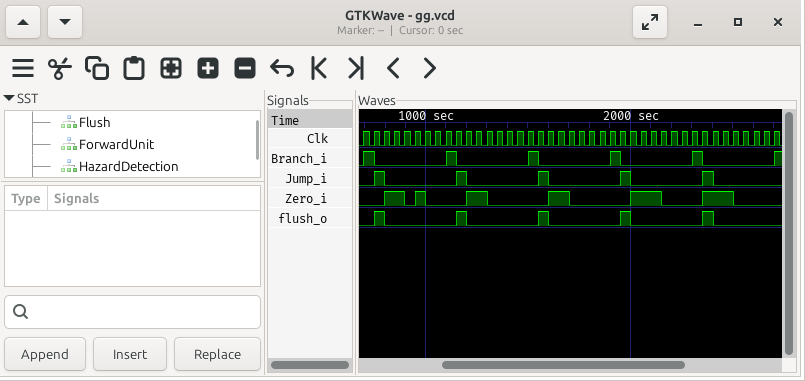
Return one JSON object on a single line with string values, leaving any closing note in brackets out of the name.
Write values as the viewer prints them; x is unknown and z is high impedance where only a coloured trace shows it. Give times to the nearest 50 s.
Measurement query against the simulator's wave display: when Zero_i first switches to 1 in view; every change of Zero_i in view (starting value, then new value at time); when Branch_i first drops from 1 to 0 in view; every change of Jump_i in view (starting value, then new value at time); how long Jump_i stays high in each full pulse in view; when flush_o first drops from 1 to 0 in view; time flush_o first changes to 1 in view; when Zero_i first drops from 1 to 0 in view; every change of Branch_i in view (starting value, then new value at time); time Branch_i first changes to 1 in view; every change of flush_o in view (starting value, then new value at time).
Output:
{"when Zero_i first switches to 1 in view": "800 s", "every change of Zero_i in view": "0, 1 at 800 s, 0 at 900 s, 1 at 950 s, 0 at 1000 s, 1 at 1200 s, 0 at 1300 s, 1 at 1600 s, 0 at 1700 s, 1 at 2000 s, 0 at 2150 s, 1 at 2350 s, 0 at 2500 s", "when Branch_i first drops from 1 to 0 in view": "750 s", "every change of Jump_i in view": "0, 1 at 750 s, 0 at 800 s, 1 at 1150 s, 0 at 1200 s, 1 at 1550 s, 0 at 1600 s, 1 at 1950 s, 0 at 2000 s, 1 at 2350 s, 0 at 2400 s", "how long Jump_i stays high in each full pulse in view": "50 s, 50 s, 50 s, 50 s, 50 s", "when flush_o first drops from 1 to 0 in view": "800 s", "time flush_o first changes to 1 in view": "750 s", "when Zero_i first drops from 1 to 0 in view": "900 s", "every change of Branch_i in view": "0, 1 at 700 s, 0 at 750 s, 1 at 1100 s, 0 at 1150 s, 1 at 1500 s, 0 at 1550 s, 1 at 1900 s, 0 at 1950 s, 1 at 2300 s, 0 at 2350 s, 1 at 2700 s", "time Branch_i first changes to 1 in view": "700 s", "every change of flush_o in view": "0, 1 at 750 s, 0 at 800 s, 1 at 1150 s, 0 at 1200 s, 1 at 1550 s, 0 at 1600 s, 1 at 1950 s, 0 at 2000 s, 1 at 2350 s, 0 at 2400 s"}
